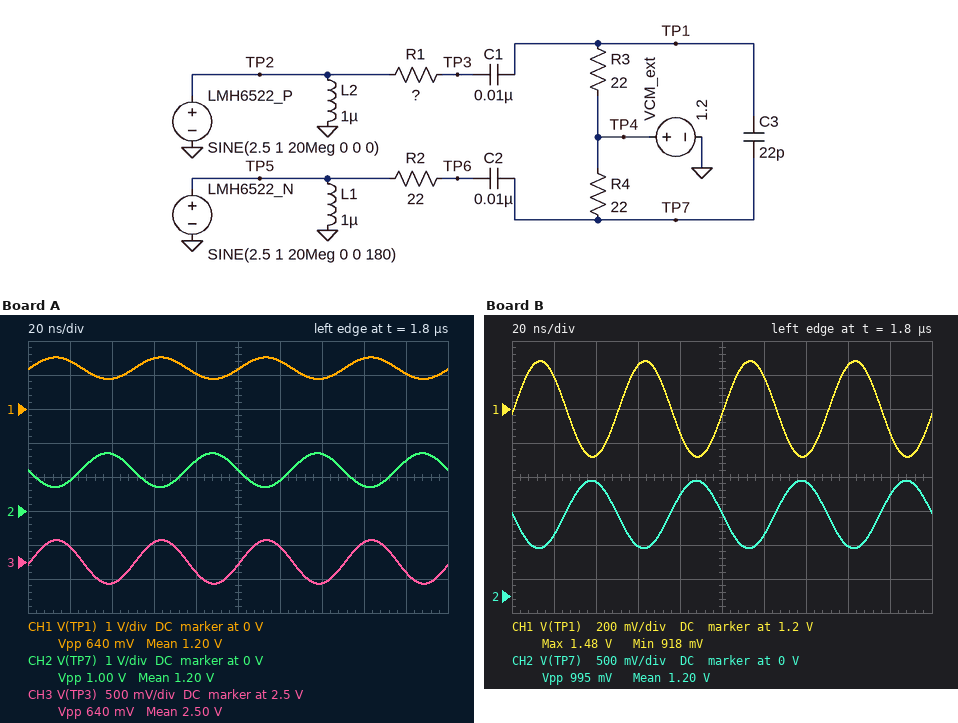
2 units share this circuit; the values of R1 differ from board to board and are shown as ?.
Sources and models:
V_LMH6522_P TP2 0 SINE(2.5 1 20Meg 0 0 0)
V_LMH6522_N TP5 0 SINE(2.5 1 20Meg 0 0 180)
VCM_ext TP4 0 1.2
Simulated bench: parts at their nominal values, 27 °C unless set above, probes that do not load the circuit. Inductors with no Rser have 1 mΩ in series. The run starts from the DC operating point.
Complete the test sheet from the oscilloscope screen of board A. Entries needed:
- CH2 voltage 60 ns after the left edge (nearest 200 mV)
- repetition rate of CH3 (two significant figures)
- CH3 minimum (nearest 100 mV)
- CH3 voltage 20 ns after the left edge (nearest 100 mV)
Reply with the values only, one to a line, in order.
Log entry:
800 mV
20 MHz
2.2 V
2.7 V
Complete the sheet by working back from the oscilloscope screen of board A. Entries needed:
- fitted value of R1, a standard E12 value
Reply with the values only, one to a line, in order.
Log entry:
47 Ω
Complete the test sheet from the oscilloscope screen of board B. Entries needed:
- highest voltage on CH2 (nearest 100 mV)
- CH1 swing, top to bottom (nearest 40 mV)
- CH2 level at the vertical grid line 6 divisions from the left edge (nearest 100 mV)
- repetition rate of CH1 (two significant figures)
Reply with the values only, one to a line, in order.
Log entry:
1.7 V
560 mV
900 mV
20 MHz
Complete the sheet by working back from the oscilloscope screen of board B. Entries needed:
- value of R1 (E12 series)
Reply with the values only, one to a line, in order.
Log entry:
56 Ω
